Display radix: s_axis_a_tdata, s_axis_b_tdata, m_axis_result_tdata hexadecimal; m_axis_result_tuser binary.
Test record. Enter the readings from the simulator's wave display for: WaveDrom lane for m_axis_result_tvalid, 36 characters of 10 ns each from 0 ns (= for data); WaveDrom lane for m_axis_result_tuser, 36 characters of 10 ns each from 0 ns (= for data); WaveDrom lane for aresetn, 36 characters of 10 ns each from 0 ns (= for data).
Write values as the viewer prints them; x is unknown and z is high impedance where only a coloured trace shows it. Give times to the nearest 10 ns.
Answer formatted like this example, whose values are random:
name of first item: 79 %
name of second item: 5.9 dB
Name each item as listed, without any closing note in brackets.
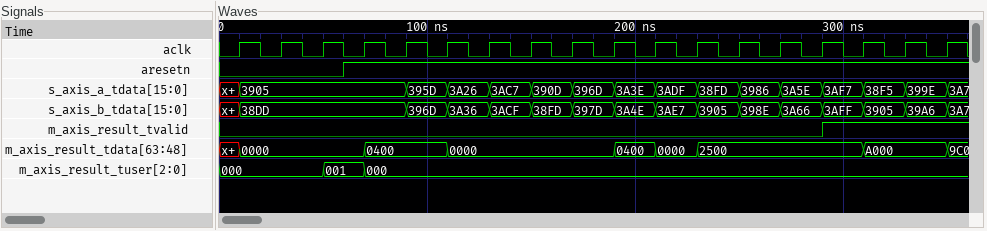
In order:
WaveDrom lane for m_axis_result_tvalid, 36 characters of 10 ns each from 0 ns: {name: 'm_axis_result_tvalid', wave: '0............................1......'}
WaveDrom lane for m_axis_result_tuser, 36 characters of 10 ns each from 0 ns: {name: 'm_axis_result_tuser', wave: '=....=.=............................', data: '000 001 000'}
WaveDrom lane for aresetn, 36 characters of 10 ns each from 0 ns: {name: 'aresetn', wave: '0.....1.............................'}
